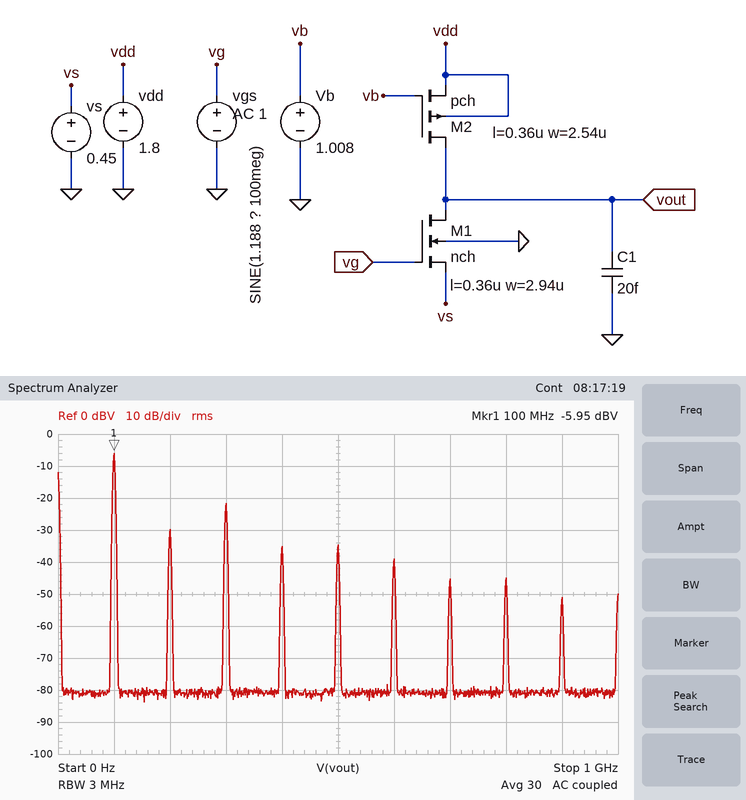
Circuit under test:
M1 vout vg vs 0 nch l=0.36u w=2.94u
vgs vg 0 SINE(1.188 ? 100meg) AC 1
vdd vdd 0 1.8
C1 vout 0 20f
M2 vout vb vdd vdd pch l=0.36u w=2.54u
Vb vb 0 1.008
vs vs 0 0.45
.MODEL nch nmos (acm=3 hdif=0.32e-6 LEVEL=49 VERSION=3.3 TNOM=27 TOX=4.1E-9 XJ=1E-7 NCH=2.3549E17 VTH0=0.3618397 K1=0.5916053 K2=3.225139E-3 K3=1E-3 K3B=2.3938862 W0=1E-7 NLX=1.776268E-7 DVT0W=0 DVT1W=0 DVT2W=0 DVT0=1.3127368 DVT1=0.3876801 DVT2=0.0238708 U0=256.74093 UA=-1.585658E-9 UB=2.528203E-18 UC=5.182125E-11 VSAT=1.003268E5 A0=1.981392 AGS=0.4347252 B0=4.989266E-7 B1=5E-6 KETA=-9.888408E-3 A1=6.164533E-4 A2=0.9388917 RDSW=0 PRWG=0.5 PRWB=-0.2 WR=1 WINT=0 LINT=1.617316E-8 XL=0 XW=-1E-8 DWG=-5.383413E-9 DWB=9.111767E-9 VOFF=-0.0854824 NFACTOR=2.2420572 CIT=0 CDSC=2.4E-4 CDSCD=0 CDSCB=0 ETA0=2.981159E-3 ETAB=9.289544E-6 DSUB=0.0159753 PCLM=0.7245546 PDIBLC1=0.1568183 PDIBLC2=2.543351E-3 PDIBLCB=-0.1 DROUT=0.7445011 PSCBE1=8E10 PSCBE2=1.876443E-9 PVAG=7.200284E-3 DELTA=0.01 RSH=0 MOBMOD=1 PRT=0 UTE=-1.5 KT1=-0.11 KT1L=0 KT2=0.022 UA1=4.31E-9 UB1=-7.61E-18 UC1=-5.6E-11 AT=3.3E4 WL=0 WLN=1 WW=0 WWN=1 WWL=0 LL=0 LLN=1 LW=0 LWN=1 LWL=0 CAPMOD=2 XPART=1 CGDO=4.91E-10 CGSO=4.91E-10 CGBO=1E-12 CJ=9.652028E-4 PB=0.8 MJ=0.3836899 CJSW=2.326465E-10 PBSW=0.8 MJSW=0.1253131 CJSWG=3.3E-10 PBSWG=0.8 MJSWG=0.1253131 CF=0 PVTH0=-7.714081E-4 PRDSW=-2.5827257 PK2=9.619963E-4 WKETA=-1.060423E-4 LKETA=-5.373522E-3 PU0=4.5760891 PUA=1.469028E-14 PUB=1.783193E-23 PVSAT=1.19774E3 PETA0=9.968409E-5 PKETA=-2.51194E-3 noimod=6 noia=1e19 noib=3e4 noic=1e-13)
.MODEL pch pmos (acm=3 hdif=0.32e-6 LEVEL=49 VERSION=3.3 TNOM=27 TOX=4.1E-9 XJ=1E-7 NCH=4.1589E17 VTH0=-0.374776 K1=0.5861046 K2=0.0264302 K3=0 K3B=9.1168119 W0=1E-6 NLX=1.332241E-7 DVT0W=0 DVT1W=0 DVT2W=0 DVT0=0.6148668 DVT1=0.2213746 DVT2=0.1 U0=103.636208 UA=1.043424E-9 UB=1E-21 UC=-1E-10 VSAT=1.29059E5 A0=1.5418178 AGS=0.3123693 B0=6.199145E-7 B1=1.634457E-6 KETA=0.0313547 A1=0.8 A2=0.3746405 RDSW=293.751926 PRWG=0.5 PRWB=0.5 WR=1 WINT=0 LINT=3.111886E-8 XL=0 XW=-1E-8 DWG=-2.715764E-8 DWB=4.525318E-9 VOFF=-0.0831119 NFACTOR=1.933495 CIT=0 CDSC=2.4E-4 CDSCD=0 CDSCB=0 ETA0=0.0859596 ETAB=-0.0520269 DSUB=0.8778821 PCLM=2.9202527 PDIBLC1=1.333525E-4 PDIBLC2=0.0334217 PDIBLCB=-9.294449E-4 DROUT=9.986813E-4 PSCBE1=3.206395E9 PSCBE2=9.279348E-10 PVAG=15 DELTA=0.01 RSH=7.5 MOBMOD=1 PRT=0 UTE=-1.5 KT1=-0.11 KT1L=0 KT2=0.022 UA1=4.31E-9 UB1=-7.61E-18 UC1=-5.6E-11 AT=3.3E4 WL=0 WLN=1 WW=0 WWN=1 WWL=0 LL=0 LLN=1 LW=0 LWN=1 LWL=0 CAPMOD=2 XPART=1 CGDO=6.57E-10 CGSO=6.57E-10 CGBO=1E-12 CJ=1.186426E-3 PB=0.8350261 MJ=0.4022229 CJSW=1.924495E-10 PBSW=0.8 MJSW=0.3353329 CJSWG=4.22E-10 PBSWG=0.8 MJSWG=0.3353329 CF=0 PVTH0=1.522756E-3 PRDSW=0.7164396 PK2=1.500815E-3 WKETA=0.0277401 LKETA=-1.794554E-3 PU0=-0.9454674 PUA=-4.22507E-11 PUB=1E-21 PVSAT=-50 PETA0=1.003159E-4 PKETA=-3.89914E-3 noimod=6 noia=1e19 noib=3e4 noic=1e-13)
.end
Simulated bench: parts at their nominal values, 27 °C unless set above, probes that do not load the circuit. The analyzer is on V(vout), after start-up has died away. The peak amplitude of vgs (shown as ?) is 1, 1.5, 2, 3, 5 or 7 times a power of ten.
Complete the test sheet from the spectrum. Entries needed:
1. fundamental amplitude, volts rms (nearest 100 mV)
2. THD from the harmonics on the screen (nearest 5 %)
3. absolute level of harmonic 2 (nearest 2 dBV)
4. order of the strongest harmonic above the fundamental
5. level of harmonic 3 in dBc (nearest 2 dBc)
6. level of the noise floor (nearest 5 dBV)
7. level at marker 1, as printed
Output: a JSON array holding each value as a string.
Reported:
["500 mV", "20 %", "-30 dBV", "3", "-16 dBc", "-80 dBV", "-5.95 dBV"]
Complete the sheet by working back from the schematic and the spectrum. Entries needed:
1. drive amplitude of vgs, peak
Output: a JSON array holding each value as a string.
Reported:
["100 mV"]
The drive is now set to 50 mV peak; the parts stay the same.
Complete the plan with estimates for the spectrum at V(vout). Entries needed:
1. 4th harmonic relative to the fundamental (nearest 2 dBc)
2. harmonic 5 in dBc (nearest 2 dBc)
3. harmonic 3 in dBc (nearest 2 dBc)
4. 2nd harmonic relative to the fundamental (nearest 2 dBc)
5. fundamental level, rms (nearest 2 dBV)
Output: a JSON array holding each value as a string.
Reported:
["-34 dBc", "-36 dBc", "-20 dBc", "-30 dBc", "-8 dBV"]
